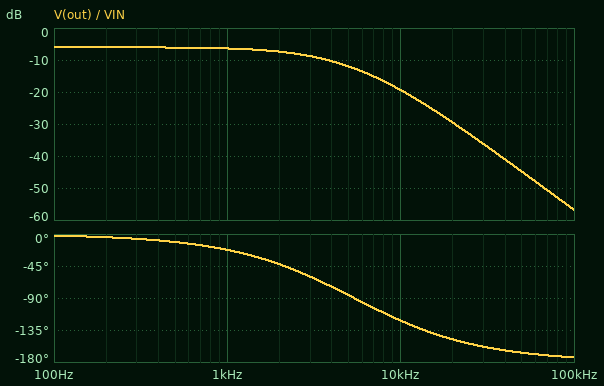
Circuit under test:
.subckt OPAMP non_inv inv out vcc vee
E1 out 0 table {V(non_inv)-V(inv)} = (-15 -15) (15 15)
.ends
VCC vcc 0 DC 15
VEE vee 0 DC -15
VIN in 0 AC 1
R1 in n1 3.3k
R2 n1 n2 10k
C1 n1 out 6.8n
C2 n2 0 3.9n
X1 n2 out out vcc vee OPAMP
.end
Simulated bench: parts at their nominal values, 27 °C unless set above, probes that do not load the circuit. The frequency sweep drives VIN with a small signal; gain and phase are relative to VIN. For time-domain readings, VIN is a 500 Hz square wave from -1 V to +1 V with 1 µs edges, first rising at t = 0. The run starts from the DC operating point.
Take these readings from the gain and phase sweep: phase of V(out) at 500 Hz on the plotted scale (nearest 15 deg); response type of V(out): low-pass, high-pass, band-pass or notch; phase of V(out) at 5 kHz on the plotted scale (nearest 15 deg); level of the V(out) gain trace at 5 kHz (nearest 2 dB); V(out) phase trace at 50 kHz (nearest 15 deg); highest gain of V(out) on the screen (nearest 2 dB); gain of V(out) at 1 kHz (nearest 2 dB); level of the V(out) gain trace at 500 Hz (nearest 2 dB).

-15 deg
low-pass
-90 deg
-12 dB
-165 deg
-6 dB
-6 dB
-6 dB
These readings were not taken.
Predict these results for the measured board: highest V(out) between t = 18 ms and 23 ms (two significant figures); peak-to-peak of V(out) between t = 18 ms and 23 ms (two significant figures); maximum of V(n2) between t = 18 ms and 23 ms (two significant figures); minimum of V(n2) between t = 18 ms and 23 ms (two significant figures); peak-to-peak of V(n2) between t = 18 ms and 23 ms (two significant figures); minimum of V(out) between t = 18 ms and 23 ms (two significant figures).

500 mV
1.0 V
1.0 V
-1.0 V
2.0 V
-500 mV
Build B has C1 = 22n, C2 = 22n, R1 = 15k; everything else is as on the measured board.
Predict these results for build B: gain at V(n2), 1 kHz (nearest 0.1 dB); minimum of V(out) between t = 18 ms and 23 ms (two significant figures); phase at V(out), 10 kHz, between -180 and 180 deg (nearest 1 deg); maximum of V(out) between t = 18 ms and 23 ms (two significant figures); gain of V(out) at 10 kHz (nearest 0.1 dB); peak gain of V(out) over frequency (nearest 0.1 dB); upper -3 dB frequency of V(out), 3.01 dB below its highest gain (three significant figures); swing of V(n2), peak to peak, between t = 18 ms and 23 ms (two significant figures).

-13.7 dB
-310 mV
-171 deg
310 mV
-55.2 dB
-6.0 dB
258 Hz
1.2 V
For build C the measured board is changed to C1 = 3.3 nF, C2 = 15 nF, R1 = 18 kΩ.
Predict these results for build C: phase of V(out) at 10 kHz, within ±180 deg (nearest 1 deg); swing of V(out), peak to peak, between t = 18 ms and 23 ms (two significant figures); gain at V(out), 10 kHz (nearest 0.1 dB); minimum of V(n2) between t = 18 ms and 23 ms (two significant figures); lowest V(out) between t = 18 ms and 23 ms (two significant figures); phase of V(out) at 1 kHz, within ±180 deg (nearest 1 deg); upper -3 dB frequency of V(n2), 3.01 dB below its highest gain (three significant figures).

-140 deg
810 mV
-39.0 dB
-810 mV
-410 mV
-77 deg
370 Hz
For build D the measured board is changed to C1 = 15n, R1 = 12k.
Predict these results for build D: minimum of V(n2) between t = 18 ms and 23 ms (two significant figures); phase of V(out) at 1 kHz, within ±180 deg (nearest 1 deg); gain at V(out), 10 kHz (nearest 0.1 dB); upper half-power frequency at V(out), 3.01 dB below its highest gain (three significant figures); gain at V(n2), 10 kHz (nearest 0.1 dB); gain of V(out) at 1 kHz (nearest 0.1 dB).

-1.0 V
-57 deg
-35.2 dB
1.14 kHz
-29.2 dB
-8.4 dB
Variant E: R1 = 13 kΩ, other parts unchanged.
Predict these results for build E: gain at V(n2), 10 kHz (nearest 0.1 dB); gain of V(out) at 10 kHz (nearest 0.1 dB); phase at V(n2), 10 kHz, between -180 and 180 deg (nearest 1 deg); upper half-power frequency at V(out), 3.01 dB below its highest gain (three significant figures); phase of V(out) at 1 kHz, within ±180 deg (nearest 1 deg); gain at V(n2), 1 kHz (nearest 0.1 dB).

-23.6 dB
-29.6 dB
-146 deg
1.45 kHz
-44 deg
-1.6 dB
